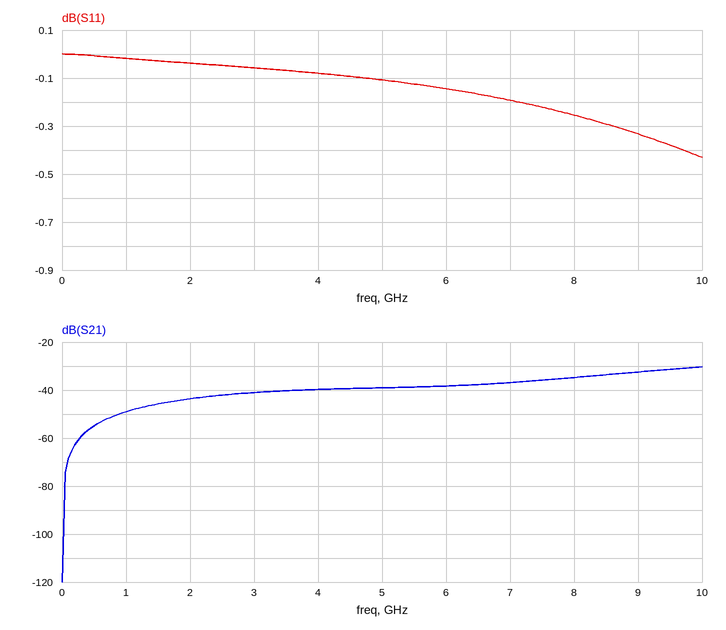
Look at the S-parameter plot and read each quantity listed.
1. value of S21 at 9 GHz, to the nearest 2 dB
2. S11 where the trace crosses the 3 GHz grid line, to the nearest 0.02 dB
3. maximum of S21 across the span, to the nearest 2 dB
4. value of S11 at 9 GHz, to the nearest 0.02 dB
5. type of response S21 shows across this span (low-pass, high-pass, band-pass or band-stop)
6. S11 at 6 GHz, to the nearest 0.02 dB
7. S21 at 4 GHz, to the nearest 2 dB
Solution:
-32 dB
-0.06 dB
-30 dB
-0.34 dB
high-pass
-0.14 dB
-40 dB
